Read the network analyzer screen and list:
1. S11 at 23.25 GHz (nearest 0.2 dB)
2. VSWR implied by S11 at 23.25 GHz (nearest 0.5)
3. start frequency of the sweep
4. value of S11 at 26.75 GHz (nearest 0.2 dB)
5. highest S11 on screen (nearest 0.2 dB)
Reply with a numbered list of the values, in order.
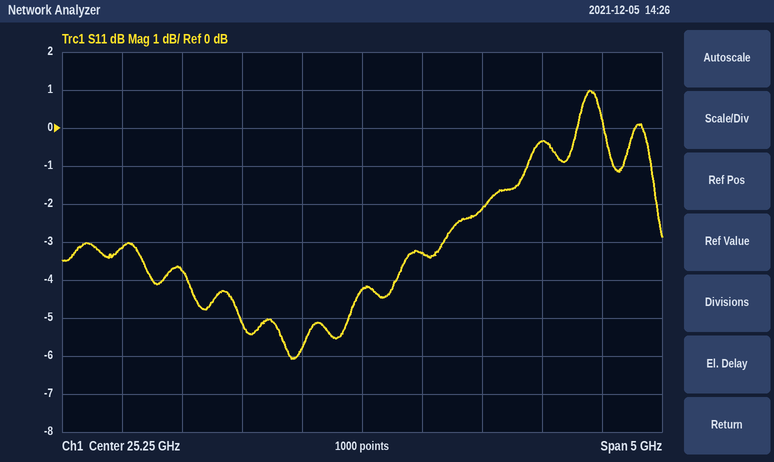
1. -3.2 dB
2. 5.5
3. 22.75 GHz
4. -0.4 dB
5. 1.0 dB
